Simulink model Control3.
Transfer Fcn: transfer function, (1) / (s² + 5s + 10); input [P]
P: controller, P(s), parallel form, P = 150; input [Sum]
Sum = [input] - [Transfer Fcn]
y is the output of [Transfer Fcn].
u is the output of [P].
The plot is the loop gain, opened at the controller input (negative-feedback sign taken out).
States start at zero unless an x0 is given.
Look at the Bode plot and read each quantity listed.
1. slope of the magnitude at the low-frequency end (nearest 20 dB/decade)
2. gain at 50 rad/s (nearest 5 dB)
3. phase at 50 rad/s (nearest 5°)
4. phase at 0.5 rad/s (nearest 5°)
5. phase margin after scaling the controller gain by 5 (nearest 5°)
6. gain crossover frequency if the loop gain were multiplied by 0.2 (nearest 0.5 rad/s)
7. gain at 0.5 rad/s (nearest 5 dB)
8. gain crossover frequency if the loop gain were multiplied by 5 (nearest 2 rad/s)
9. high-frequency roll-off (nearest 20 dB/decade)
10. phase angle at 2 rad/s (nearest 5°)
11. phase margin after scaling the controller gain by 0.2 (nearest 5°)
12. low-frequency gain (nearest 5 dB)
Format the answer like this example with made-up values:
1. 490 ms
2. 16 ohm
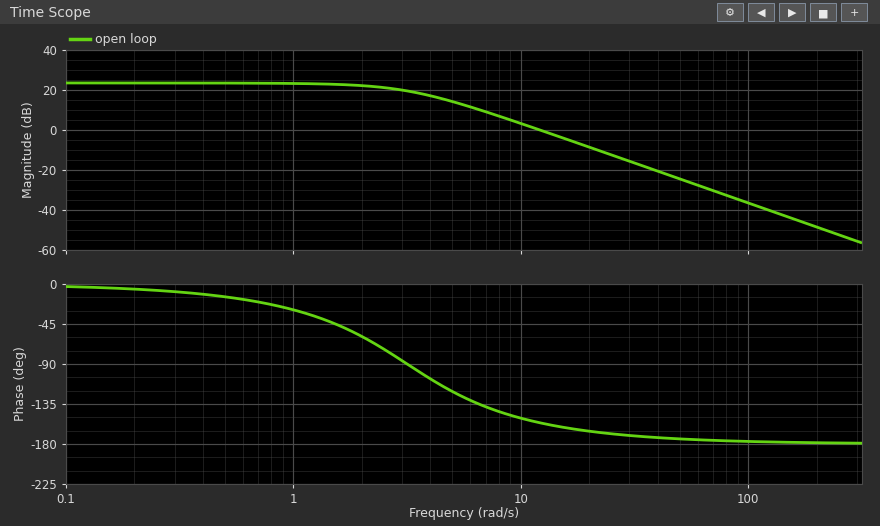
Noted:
1. 0 dB/decade
2. -25 dB
3. -175°
4. -15°
5. 10°
6. 5.0 rad/s
7. 25 dB
8. 28 rad/s
9. -40 dB/decade
10. -60°
11. 60°
12. 25 dB
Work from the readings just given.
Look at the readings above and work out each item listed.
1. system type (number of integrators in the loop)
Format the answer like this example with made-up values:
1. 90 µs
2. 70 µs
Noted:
1. 0
